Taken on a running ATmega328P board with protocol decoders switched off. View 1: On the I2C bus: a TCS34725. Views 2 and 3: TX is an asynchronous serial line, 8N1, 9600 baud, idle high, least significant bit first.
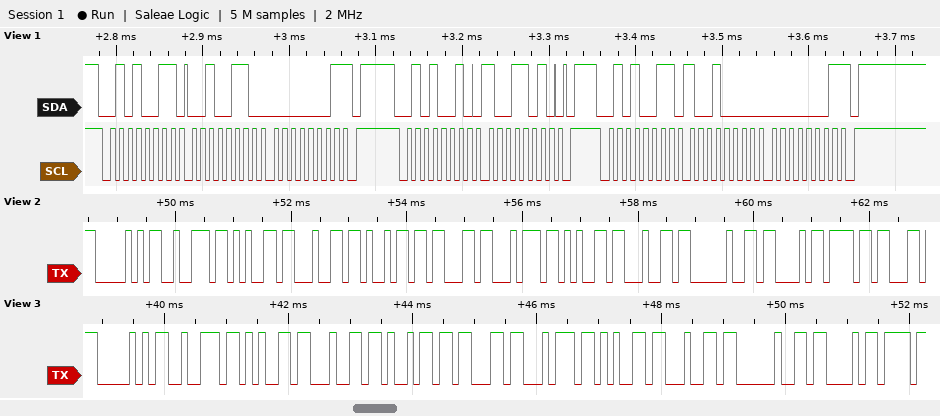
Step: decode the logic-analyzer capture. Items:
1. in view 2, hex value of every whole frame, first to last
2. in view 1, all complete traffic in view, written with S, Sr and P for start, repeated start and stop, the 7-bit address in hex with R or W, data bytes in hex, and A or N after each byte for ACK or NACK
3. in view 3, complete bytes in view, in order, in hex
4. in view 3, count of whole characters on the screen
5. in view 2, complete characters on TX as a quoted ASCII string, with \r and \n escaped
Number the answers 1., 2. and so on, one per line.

1. 50 72 65 64 69 63 74 65 64 20 43 6F
2. S 29R A 26 A 01 N P S 29W A 9A A P S 29R A 90 A 01 N P
3. 50 72 65 64 69 63 74 65 64 20 43
4. 11
5. "Predicted Co"
